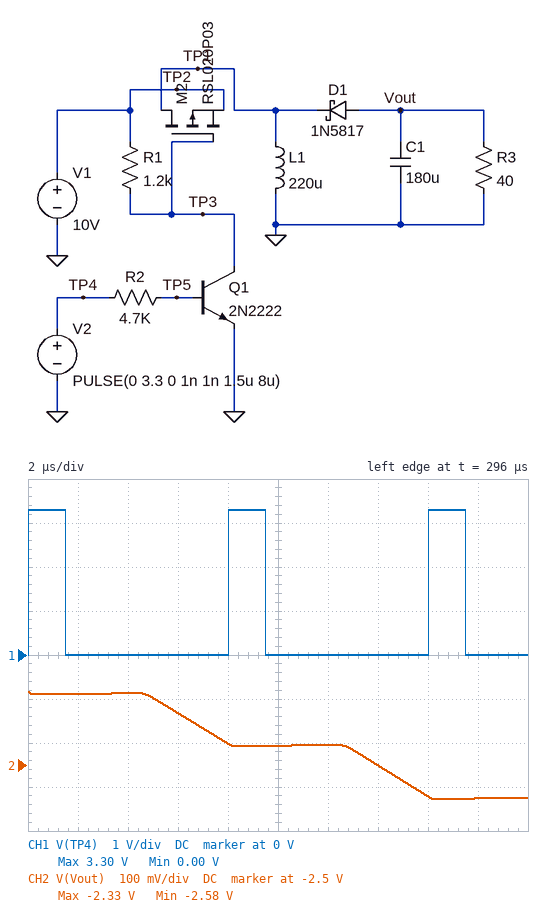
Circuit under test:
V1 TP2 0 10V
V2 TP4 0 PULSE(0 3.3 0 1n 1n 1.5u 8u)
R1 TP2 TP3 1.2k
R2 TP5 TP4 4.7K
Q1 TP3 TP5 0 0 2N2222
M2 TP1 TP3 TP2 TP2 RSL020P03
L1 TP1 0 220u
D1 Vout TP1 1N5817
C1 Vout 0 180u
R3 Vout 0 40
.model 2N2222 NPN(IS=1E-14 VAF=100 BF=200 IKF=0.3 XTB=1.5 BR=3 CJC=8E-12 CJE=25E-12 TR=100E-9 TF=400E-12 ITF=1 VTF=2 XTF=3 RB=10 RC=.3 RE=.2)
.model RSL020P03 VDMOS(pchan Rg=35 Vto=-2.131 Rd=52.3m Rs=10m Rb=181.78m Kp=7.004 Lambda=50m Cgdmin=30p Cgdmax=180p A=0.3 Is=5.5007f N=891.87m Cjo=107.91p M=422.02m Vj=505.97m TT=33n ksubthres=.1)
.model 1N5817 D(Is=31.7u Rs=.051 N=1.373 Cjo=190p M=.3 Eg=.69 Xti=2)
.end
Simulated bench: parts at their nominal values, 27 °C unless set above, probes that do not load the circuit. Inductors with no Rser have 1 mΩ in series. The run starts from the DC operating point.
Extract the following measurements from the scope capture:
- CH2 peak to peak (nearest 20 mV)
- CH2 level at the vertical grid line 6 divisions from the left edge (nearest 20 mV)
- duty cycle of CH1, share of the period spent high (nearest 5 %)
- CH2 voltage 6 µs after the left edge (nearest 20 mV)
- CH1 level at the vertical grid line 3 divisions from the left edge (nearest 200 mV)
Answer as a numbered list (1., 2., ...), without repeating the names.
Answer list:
1. 240 mV
2. -2.46 V
3. 20 %
4. -2.38 V
5. 0 V
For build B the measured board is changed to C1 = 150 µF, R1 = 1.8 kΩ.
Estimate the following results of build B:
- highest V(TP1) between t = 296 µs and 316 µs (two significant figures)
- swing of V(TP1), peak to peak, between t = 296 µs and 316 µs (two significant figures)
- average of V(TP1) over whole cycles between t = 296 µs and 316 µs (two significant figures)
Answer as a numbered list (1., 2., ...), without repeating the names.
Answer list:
1. 9.3 V
2. 13 V
3. 4.7 V
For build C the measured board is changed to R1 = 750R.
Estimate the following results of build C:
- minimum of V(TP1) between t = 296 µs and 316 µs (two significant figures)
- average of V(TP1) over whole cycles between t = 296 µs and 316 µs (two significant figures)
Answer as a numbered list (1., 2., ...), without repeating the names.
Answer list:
1. -3.2 V
2. 2.1 V
